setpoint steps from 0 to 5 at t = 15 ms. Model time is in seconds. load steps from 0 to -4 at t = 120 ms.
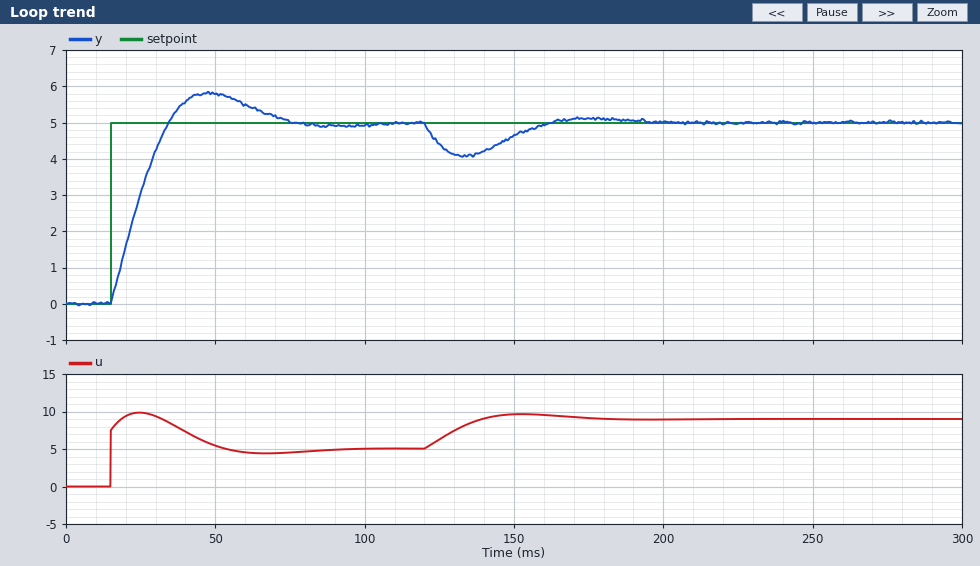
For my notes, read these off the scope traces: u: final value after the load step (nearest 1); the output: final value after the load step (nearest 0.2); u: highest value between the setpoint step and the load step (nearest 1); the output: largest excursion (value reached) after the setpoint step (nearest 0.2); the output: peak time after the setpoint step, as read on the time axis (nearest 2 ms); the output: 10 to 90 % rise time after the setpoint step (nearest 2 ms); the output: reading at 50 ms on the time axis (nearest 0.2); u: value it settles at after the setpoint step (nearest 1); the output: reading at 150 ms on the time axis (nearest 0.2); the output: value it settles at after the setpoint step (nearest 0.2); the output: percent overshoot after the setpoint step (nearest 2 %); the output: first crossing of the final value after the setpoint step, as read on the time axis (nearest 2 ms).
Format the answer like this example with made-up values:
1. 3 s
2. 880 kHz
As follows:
1. 9
2. 5.0
3. 10
4. 5.8
5. 48 ms
6. 14 ms
7. 5.8
8. 5
9. 4.6
10. 5.0
11. 16 %
12. 34 ms
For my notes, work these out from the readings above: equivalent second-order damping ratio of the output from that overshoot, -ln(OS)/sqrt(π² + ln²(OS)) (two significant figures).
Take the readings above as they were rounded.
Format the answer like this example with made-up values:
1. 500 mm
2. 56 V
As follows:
1. 0.50
